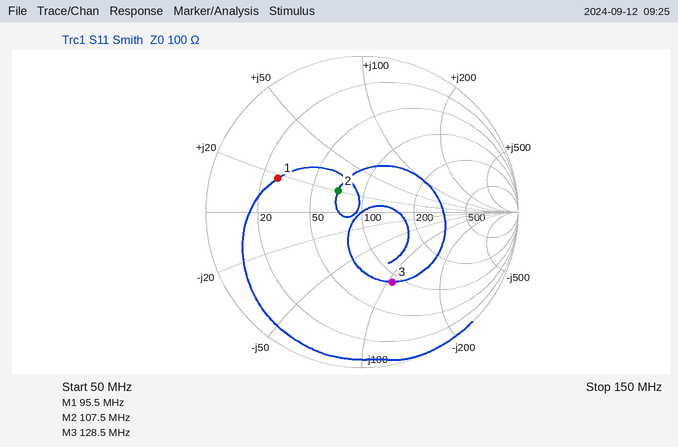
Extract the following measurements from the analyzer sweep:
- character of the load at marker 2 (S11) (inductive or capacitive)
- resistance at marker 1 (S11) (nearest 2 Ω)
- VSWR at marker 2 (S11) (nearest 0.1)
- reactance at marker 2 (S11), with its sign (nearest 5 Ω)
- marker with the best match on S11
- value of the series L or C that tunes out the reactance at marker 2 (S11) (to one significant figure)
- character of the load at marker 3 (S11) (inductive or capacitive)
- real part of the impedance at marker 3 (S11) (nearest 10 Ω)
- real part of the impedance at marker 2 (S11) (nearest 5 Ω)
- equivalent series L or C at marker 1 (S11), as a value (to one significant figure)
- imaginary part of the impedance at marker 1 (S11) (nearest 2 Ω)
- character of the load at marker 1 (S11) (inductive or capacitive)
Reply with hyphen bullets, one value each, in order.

- inductive
- 28 Ω
- 1.5
- +20 Ω
- marker 2
- 70 pF
- capacitive
- 90 Ω
- 70 Ω
- 30 nH
- +18 Ω
- inductive
